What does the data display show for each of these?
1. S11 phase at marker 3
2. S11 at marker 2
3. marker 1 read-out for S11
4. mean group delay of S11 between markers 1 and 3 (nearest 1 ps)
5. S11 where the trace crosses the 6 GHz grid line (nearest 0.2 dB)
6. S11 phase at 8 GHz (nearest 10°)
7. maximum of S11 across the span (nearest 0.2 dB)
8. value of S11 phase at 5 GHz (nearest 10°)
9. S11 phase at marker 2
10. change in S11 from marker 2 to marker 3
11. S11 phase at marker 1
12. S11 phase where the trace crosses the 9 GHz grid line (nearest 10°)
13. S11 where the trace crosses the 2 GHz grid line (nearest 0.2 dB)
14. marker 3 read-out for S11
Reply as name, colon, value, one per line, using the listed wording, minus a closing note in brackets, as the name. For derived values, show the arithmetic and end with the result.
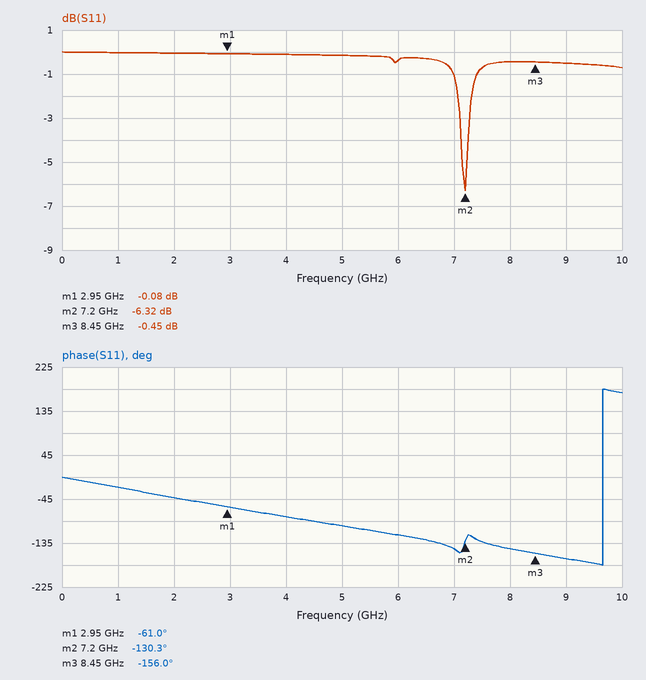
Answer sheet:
S11 phase at marker 3: -156.0°
S11 at marker 2: -6.32 dB
marker 1 read-out for S11: -0.08 dB
mean group delay of S11 between markers 1 and 3: −(-156° − (-61°))/(360° × 5.5 GHz) ≈ 48 ps
S11 where the trace crosses the 6 GHz grid line: -0.4 dB
S11 phase at 8 GHz: -150°
maximum of S11 across the span: 0.0 dB
value of S11 phase at 5 GHz: -100°
S11 phase at marker 2: -130.3°
change in S11 from marker 2 to marker 3: -0.45 − (-6.32) = 5.87 dB
S11 phase at marker 1: -61.0°
S11 phase where the trace crosses the 9 GHz grid line: -170°
S11 where the trace crosses the 2 GHz grid line: 0.0 dB
marker 3 read-out for S11: -0.45 dB
